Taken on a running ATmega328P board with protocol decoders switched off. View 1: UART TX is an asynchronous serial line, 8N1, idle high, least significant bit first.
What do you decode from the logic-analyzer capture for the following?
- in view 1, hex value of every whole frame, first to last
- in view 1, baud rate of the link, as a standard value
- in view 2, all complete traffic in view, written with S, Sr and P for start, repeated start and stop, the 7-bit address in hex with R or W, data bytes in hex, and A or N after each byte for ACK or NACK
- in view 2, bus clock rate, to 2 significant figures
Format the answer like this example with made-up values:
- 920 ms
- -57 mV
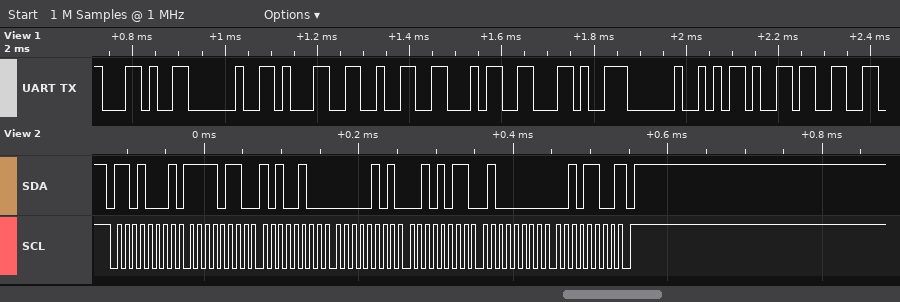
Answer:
- 2C 20 31 32 34 2C 20 2D 33
- 57600 baud
- S 68R A F6 A A4 A 05 A 2B A 40 A 2C N P
- 100 kHz
